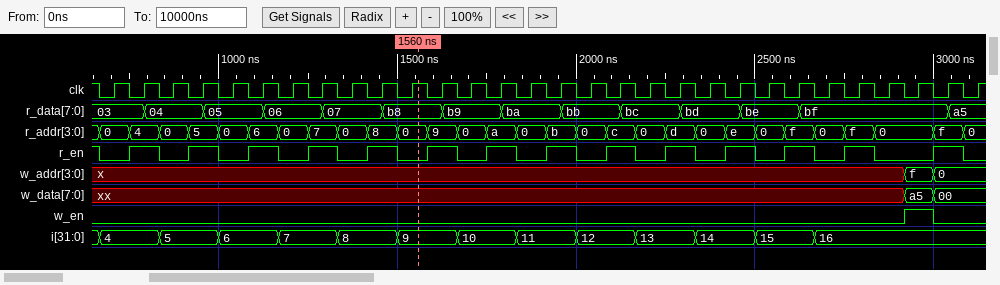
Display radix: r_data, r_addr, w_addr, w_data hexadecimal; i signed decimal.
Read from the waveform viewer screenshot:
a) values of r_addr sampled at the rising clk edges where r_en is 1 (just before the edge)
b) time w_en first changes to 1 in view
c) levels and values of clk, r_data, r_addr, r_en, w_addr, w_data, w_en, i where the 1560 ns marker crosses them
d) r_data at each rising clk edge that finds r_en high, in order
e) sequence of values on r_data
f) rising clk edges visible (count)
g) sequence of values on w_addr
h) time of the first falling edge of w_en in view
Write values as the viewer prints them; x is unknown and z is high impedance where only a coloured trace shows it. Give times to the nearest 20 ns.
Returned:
4, 5, 6, 7, 8, 9, a, b, c, d, e, f, f, f
2920 ns
clk=1, r_data=b8, r_addr=0, r_en=0, w_addr=x, w_data=xx, w_en=0, i=9
03, 04, 05, 06, 07, b8, b9, ba, bb, bc, bd, be, bf, bf
03, 04, 05, 06, 07, b8, b9, ba, bb, bc, bd, be, bf, a5
30
x, f, 0
3000 ns
